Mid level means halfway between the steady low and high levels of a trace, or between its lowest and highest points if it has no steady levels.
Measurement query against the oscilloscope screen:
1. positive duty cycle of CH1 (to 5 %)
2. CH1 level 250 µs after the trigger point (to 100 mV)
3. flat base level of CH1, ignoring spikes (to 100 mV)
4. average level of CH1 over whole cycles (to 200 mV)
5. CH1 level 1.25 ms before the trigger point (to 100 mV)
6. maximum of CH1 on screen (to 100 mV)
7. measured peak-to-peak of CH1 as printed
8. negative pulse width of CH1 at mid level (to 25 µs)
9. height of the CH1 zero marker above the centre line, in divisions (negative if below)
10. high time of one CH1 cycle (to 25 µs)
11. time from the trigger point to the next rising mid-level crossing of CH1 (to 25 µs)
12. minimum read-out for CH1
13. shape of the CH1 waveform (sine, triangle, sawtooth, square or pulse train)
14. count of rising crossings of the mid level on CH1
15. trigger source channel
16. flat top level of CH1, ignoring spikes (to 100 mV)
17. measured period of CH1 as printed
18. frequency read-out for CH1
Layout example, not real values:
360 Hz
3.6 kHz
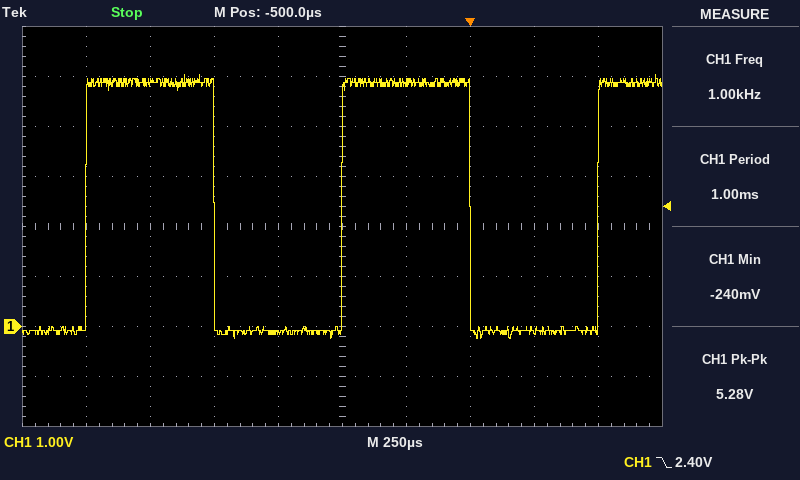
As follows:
50 %
-100 mV
-100 mV
2.4 V
4.9 V
5.0 V
5.28 V
500 µs
-2.0 div
500 µs
500 µs
-240 mV
square
3
CH1
4.9 V
1.00 ms
1.00 kHz
